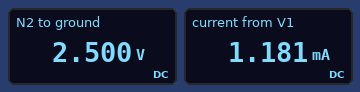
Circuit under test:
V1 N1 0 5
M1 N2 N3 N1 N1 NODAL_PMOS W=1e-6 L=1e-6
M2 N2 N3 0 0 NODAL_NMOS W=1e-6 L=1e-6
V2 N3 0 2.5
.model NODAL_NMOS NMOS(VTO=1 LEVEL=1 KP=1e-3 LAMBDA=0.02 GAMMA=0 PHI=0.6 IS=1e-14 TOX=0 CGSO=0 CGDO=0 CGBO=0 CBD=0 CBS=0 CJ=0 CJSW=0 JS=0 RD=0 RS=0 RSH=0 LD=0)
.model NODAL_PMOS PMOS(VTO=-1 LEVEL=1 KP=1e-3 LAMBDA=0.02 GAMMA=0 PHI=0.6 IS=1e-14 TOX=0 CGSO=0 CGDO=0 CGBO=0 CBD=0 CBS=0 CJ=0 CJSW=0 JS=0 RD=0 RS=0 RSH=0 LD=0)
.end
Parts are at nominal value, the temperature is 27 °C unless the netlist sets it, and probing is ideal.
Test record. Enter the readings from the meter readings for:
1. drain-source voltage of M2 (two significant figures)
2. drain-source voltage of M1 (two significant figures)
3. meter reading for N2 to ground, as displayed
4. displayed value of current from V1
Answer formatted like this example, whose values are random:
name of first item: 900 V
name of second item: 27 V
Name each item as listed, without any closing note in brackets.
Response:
drain-source voltage of M2: 2.5 V
drain-source voltage of M1: -2.5 V
meter reading for N2 to ground, as displayed: 2.500 V
displayed value of current from V1: 1.181 mA
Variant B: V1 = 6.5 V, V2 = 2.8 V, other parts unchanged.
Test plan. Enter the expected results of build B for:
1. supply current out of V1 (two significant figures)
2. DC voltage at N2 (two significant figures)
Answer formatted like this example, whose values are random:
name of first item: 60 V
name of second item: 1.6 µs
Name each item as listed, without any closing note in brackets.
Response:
supply current out of V1: 1.8 mA
DC voltage at N2: 5.7 V
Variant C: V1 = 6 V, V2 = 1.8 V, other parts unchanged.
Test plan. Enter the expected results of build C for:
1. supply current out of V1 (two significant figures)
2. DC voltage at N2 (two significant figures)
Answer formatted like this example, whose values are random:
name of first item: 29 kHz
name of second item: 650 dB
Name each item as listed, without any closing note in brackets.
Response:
supply current out of V1: 360 µA
DC voltage at N2: 5.9 V
